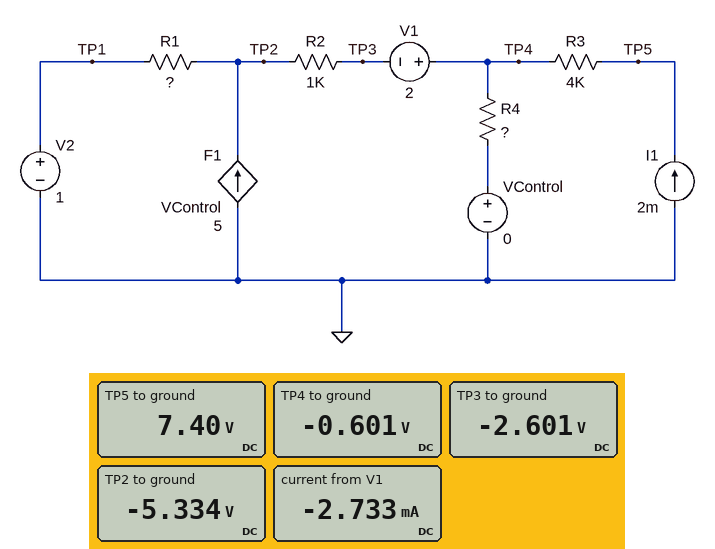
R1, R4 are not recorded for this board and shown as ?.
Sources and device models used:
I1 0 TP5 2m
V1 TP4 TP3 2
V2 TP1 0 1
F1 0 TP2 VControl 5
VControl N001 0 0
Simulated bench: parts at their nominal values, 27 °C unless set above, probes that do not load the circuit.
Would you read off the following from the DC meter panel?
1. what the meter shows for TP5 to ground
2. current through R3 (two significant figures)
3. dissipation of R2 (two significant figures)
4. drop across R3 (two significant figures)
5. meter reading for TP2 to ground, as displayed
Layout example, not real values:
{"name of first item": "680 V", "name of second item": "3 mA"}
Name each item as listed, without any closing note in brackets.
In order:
{"what the meter shows for TP5 to ground": "7.40 V", "current through R3": "2.0 mA", "dissipation of R2": "7.5 mW", "drop across R3": "8.0 V", "meter reading for TP2 to ground, as displayed": "-5.334 V"}
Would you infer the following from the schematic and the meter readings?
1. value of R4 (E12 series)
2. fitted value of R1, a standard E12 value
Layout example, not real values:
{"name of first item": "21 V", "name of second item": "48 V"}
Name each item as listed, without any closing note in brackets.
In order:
{"value of R4": "820 Ω", "fitted value of R1, a standard E12 value": "6.8 kΩ"}
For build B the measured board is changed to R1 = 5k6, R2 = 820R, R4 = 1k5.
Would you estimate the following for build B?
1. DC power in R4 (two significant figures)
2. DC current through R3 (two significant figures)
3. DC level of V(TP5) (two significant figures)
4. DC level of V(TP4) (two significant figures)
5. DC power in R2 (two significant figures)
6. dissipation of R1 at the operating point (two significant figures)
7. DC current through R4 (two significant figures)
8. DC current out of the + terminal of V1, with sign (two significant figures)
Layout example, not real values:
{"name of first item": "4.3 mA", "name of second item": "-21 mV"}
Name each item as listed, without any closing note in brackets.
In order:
{"DC power in R4": "930 µW", "DC current through R3": "2.0 mA", "DC level of V(TP5)": "6.8 V", "DC level of V(TP4)": "-1.2 V", "DC power in R2": "6.4 mW", "dissipation of R1 at the operating point": "7.5 mW", "DC current through R4": "790 µA", "DC current out of the + terminal of V1, with sign": "-2.8 mA"}
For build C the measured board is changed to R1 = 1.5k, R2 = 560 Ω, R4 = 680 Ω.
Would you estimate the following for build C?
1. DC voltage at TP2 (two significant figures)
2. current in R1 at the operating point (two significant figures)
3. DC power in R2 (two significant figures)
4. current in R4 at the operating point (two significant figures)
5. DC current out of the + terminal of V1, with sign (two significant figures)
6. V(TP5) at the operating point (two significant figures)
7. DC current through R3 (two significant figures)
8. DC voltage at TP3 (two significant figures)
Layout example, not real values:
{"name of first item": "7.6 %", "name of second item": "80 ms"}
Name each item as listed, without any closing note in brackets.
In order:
{"DC voltage at TP2": "-5.0 V", "current in R1 at the operating point": "4.0 mA", "DC power in R2": "6.8 mW", "current in R4 at the operating point": "1.5 mA", "DC current out of the + terminal of V1, with sign": "-3.5 mA", "V(TP5) at the operating point": "7.0 V", "DC current through R3": "2.0 mA", "DC voltage at TP3": "-3.0 V"}
